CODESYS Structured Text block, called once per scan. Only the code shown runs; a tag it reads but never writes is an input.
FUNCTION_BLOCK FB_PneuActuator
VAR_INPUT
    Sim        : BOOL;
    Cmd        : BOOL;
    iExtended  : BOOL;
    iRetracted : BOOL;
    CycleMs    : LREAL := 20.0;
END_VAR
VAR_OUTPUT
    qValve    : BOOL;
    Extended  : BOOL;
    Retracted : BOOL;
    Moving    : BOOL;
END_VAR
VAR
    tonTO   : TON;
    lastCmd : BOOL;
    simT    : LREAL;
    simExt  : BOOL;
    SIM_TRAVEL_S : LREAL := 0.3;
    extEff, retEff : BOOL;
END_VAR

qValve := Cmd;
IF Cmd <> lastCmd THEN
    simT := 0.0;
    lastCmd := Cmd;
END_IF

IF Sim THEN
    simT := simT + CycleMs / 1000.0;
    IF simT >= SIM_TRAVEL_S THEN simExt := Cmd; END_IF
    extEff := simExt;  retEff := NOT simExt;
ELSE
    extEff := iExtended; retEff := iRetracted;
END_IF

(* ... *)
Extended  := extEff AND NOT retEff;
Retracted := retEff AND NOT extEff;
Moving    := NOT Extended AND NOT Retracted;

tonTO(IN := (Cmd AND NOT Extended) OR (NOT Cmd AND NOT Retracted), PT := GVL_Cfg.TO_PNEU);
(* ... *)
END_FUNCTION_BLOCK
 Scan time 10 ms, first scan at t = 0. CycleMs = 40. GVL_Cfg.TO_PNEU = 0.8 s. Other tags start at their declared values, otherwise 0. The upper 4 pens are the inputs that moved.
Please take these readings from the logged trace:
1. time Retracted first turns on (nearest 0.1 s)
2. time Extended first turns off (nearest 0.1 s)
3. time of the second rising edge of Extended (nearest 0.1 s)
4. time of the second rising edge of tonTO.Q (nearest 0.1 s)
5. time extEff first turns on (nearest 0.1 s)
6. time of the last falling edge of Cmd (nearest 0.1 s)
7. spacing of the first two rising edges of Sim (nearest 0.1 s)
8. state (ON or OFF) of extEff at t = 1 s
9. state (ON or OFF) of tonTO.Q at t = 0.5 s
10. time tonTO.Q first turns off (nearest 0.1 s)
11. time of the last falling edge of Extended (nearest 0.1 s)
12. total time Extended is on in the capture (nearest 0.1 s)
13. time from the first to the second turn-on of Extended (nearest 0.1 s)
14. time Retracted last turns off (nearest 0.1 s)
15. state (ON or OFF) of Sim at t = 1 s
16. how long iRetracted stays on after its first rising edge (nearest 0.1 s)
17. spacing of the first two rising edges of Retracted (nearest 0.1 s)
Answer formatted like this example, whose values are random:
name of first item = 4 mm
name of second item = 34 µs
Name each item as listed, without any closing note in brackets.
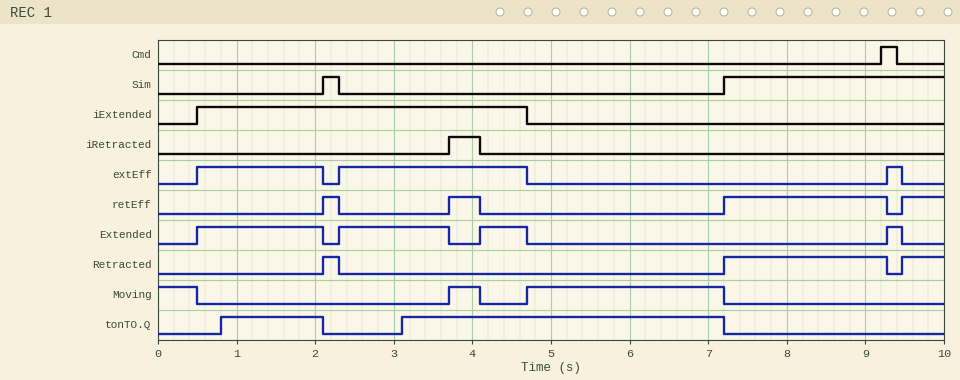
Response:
time Retracted first turns on = 2.1 s
time Extended first turns off = 2.1 s
time of the second rising edge of Extended = 2.3 s
time of the second rising edge of tonTO.Q = 3.1 s
time extEff first turns on = 0.5 s
time of the last falling edge of Cmd = 9.4 s
spacing of the first two rising edges of Sim = 5.1 s
state (ON or OFF) of extEff at t = 1 s = ON
state (ON or OFF) of tonTO.Q at t = 0.5 s = OFF
time tonTO.Q first turns off = 2.1 s
time of the last falling edge of Extended = 9.5 s
total time Extended is on in the capture = 3.8 s
time from the first to the second turn-on of Extended = 1.8 s
time Retracted last turns off = 9.3 s
state (ON or OFF) of Sim at t = 1 s = OFF
how long iRetracted stays on after its first rising edge = 0.4 s
spacing of the first two rising edges of Retracted = 5.1 s
